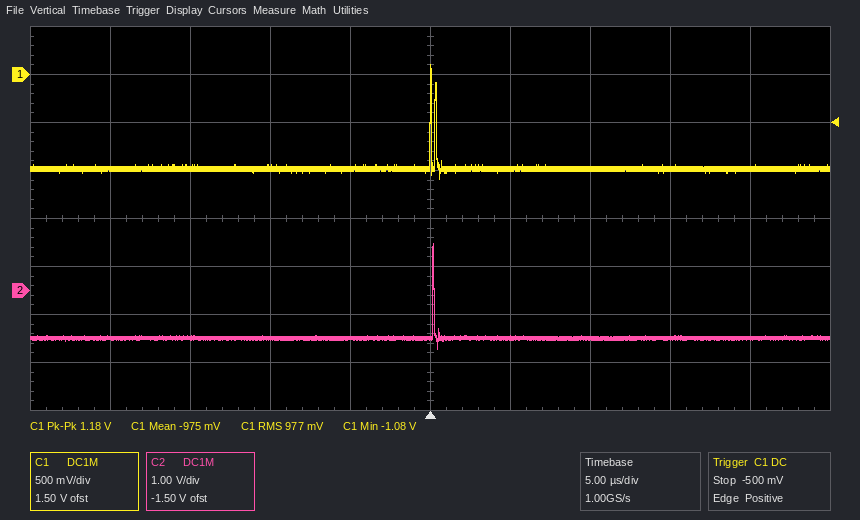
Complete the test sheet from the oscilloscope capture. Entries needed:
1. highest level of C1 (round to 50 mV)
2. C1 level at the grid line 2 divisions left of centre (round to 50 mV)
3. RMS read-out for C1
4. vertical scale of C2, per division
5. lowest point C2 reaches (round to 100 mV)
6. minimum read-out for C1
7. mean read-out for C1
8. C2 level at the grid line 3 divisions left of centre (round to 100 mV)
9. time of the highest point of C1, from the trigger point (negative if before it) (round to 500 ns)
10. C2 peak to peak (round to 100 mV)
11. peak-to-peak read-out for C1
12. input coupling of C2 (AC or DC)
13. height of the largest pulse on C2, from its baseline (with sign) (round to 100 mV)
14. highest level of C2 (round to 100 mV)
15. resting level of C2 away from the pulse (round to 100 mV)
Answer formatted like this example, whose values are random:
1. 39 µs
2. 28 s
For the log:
1. 100 mV
2. -950 mV
3. 977 mV
4. 1 V
5. -1.2 V
6. -1.08 V
7. -975 mV
8. -1.0 V
9. 0.0 µs
10. 2.2 V
11. 1.18 V
12. DC
13. +2.0 V
14. 1.0 V
15. -1.0 V
